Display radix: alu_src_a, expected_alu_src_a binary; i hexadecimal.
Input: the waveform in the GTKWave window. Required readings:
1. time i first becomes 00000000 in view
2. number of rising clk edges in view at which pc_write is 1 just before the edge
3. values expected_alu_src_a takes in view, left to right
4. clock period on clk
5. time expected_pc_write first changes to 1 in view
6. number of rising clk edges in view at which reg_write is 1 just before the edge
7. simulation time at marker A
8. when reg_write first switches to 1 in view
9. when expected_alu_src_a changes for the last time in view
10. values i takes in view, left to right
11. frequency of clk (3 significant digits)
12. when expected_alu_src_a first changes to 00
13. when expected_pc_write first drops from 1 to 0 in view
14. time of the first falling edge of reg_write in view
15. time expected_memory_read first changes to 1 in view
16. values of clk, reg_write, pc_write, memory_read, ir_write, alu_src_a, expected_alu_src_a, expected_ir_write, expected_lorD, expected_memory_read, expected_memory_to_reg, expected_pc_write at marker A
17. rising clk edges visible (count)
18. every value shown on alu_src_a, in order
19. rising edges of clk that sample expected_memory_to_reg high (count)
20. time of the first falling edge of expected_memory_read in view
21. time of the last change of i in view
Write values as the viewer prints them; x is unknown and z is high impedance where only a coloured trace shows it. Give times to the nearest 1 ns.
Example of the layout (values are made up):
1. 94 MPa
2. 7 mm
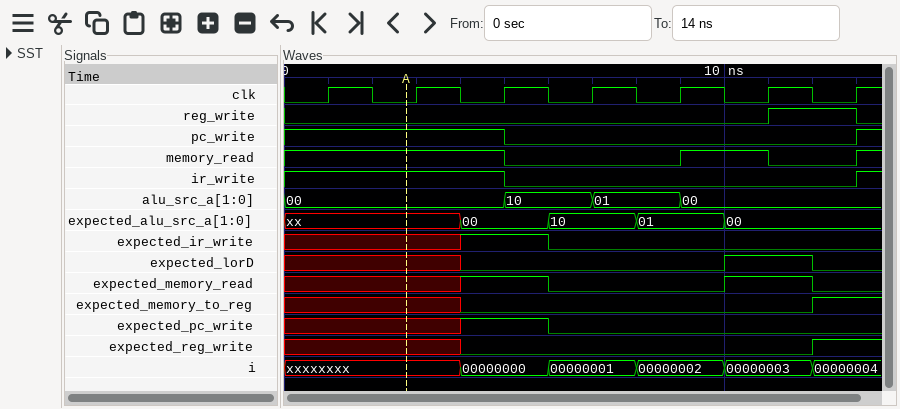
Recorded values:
1. 4 ns
2. 3
3. xx, 00, 10, 01, 00
4. 2 ns
5. 4 ns
6. 1
7. 3 ns
8. 11 ns
9. 10 ns
10. xxxxxxxx, 00000000, 00000001, 00000002, 00000003, 00000004
11. 500 MHz
12. 4 ns
13. 6 ns
14. 13 ns
15. 4 ns
16. clk=0, reg_write=0, pc_write=1, memory_read=1, ir_write=1, alu_src_a=00, expected_alu_src_a=xx, expected_ir_write=x, expected_lorD=x, expected_memory_read=x, expected_memory_to_reg=x, expected_pc_write=x
17. 7
18. 00, 10, 01, 00
19. 1
20. 6 ns
21. 12 ns
